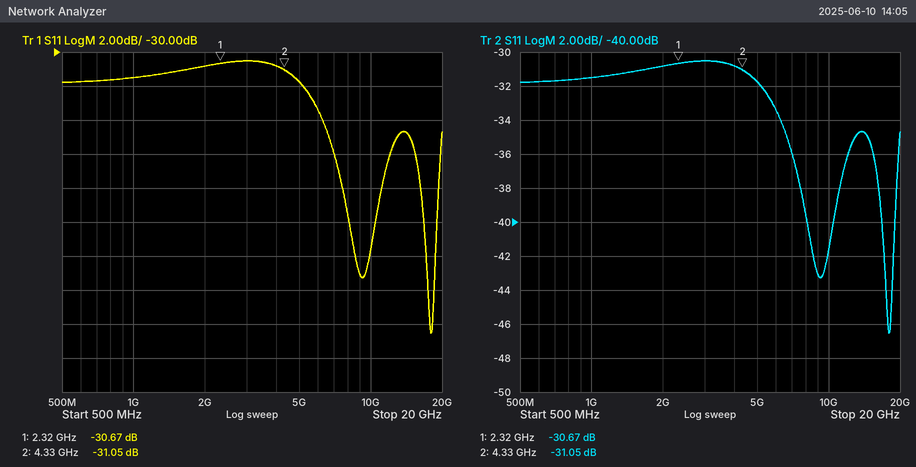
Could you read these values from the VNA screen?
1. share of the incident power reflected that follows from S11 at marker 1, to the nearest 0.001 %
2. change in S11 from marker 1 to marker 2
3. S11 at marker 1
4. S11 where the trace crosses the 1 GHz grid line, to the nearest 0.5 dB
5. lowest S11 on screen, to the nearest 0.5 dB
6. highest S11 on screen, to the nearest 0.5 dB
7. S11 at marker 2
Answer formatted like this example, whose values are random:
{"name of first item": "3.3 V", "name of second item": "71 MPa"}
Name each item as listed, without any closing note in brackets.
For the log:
{"share of the incident power reflected that follows from S11 at marker 1, to the nearest 0.001 %": "0.086 %", "change in S11 from marker 1 to marker 2": "-0.38 dB", "S11 at marker 1": "-30.67 dB", "S11 where the trace crosses the 1 GHz grid line, to the nearest 0.5 dB": "-31.5 dB", "lowest S11 on screen, to the nearest 0.5 dB": "-46.5 dB", "highest S11 on screen, to the nearest 0.5 dB": "-30.5 dB", "S11 at marker 2": "-31.05 dB"}
